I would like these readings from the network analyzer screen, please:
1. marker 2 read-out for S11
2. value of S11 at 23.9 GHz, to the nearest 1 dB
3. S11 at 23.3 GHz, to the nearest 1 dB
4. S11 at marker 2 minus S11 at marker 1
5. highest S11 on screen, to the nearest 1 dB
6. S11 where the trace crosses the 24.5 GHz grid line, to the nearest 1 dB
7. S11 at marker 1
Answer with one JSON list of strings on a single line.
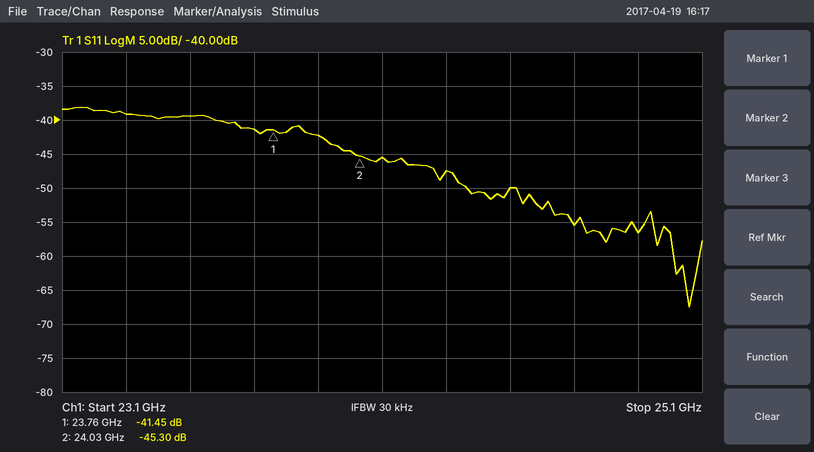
["-45.30 dB", "-42 dB", "-39 dB", "-3.85 dB", "-38 dB", "-50 dB", "-41.45 dB"]
